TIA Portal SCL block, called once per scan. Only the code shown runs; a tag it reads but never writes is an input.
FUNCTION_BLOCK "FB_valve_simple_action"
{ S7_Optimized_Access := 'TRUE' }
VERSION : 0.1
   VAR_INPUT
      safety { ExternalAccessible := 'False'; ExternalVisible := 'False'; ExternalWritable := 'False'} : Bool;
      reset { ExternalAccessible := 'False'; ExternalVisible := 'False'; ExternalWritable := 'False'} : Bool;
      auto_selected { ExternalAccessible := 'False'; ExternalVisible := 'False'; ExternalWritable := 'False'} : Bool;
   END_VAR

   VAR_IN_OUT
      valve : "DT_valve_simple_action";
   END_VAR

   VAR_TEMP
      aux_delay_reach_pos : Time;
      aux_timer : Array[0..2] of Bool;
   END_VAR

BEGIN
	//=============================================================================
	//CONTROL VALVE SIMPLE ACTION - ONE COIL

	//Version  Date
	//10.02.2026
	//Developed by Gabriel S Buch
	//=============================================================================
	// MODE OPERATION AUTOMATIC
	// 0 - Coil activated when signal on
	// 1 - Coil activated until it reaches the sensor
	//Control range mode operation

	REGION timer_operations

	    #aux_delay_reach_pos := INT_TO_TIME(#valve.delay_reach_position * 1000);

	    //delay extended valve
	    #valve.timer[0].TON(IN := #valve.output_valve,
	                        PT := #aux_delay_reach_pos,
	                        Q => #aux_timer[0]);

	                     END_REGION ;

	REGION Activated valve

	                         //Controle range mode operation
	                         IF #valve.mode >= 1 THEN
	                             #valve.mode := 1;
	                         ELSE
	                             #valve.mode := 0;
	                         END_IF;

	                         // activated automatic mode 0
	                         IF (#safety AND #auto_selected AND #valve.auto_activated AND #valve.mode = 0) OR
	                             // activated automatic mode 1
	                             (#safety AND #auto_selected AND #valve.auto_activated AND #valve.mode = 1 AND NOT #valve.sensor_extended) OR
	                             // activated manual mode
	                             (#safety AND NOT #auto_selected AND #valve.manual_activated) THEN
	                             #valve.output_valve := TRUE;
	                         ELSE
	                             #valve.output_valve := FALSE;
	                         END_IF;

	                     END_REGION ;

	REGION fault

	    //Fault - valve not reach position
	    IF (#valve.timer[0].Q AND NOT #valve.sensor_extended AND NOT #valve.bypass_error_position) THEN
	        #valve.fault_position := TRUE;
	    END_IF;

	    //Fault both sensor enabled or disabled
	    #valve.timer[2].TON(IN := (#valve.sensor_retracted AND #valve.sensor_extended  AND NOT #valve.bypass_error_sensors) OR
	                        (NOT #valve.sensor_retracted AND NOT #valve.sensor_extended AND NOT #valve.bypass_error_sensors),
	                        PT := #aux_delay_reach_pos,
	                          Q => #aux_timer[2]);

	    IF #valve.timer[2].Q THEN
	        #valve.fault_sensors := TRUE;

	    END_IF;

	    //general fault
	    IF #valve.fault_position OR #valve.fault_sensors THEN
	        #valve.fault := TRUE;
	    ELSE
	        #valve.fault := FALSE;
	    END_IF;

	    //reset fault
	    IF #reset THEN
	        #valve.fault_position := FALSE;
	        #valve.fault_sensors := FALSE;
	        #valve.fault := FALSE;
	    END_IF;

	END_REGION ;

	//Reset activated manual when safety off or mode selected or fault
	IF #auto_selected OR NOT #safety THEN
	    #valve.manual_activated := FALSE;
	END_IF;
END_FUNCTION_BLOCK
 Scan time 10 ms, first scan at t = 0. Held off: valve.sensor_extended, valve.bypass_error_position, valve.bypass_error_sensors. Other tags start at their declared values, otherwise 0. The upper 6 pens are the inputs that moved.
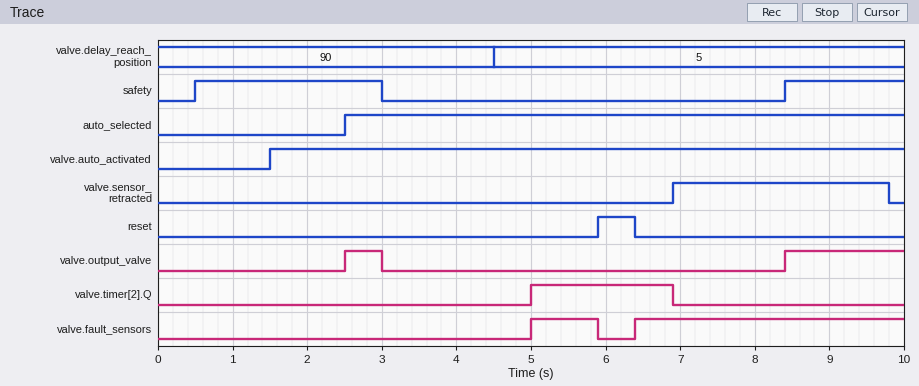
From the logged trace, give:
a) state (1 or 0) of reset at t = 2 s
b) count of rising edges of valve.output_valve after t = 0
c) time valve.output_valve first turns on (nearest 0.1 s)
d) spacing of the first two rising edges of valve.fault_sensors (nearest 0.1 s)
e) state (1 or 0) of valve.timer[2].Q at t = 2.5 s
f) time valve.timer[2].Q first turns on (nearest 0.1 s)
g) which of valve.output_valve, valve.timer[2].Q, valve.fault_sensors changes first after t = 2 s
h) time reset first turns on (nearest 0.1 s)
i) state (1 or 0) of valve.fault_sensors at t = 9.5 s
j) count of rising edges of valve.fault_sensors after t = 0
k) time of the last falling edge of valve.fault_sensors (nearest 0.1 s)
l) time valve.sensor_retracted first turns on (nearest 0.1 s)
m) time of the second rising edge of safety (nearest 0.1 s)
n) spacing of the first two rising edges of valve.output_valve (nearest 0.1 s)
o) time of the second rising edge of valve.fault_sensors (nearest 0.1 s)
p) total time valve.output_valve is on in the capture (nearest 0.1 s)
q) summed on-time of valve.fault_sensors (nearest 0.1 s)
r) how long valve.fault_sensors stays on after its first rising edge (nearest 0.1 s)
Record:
0
2
2.5 s
1.4 s
0
5.0 s
valve.output_valve
5.9 s
1
2
5.9 s
6.9 s
8.4 s
5.9 s
6.4 s
2.1 s
4.5 s
0.9 s
